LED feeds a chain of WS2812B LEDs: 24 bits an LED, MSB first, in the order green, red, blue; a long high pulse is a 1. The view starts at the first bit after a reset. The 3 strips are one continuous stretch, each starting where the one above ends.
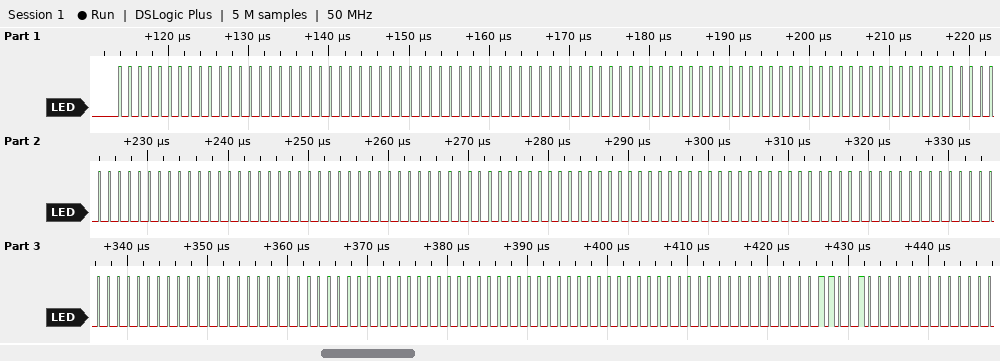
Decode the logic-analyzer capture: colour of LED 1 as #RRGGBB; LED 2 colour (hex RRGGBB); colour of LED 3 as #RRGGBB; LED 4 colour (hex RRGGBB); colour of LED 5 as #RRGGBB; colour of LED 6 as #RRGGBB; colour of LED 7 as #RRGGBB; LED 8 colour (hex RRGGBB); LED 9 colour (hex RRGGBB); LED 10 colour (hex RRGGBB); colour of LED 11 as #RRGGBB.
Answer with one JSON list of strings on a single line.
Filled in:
["#000000", "#000000", "#000000", "#000000", "#000000", "#000000", "#000000", "#000000", "#000000", "#000000", "#320000"]
